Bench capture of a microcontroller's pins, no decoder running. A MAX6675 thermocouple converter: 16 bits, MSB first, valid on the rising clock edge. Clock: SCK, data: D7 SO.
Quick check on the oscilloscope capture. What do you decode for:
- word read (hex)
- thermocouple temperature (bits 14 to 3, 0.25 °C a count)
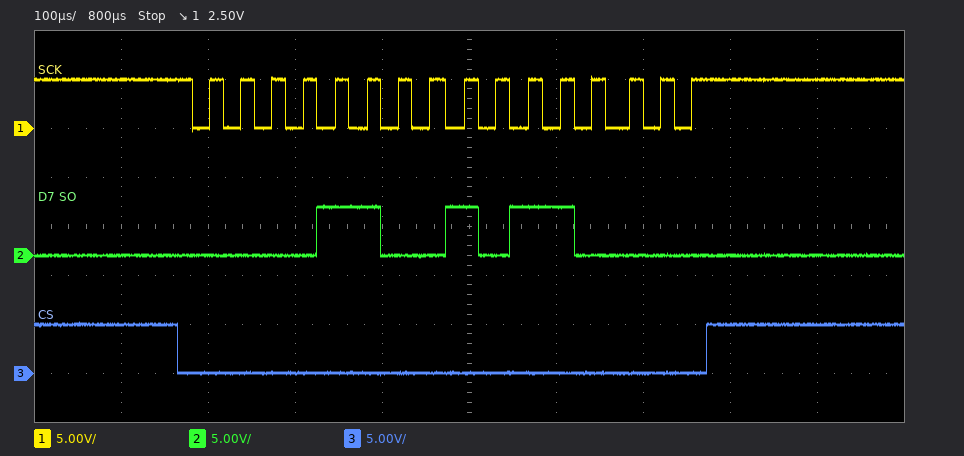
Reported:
0x0CB0
101.50 °C
